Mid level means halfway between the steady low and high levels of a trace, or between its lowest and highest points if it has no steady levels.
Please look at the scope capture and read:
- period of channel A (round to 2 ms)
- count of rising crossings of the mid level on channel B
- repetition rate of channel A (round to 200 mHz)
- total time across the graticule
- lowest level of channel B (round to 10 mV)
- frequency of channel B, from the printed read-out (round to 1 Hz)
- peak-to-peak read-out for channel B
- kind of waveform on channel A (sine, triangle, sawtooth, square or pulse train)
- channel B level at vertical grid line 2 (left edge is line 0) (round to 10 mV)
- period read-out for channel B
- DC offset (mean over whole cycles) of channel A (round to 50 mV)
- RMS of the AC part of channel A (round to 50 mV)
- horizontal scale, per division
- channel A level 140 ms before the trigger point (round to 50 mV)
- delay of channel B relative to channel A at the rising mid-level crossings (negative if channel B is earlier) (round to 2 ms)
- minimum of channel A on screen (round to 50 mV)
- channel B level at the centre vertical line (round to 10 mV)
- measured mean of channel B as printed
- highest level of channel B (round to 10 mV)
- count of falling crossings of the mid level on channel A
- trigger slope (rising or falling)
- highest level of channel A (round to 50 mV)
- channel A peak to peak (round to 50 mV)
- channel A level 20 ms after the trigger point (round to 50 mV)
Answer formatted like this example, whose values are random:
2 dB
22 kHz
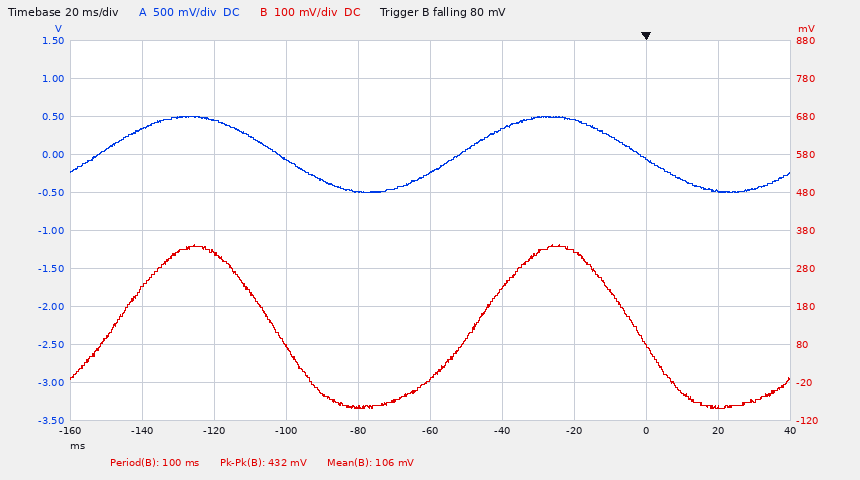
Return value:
100 ms
2
10.0 Hz
200 ms
-90 mV
10 Hz
432 mV
sine
320 mV
100 ms
0 mV
350 mV
20 ms
350 mV
+4 ms
-500 mV
-10 mV
106 mV
340 mV
2
falling
500 mV
1.00 V
-500 mV
